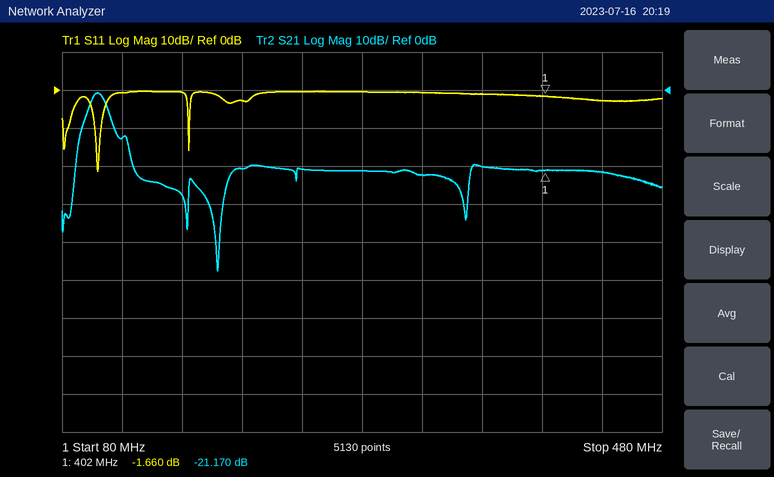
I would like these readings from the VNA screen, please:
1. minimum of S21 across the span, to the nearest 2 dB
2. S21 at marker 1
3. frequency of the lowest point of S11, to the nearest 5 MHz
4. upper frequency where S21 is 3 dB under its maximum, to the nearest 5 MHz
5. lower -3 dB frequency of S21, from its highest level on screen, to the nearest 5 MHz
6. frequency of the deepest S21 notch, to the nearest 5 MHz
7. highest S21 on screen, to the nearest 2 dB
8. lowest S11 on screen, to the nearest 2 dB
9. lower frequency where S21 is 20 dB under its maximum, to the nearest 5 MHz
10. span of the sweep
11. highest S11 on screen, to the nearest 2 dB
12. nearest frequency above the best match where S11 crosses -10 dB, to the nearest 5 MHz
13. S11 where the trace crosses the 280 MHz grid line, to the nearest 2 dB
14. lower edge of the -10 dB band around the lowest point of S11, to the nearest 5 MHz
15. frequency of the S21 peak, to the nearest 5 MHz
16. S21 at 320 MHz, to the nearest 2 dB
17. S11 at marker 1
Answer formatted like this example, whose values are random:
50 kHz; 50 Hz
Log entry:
-48 dB; -21.170 dB; 105 MHz; 110 MHz; 100 MHz; 185 MHz; 0 dB; -22 dB; 90 MHz; 400 MHz; 0 dB; 105 MHz; 0 dB; 100 MHz; 105 MHz; -22 dB; -1.660 dB
